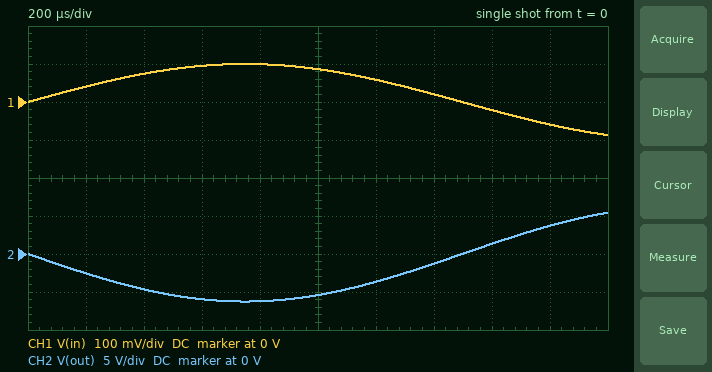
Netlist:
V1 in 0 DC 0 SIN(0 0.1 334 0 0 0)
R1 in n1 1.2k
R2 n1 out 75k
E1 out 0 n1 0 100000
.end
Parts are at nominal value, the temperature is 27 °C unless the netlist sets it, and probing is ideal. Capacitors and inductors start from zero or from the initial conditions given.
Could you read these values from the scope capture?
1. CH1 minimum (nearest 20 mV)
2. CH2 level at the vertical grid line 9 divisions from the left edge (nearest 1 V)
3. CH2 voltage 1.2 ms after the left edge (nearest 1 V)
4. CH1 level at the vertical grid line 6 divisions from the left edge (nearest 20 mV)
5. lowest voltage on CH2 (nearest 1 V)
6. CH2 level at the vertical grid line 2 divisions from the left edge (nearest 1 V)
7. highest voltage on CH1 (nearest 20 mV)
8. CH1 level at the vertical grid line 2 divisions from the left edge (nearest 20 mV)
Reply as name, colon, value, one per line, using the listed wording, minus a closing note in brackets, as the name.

CH1 minimum: -80 mV
CH2 level at the vertical grid line 9 divisions from the left edge: 4 V
CH2 voltage 1.2 ms after the left edge: -4 V
CH1 level at the vertical grid line 6 divisions from the left edge: 60 mV
lowest voltage on CH2: -6 V
CH2 level at the vertical grid line 2 divisions from the left edge: -5 V
highest voltage on CH1: 100 mV
CH1 level at the vertical grid line 2 divisions from the left edge: 80 mV
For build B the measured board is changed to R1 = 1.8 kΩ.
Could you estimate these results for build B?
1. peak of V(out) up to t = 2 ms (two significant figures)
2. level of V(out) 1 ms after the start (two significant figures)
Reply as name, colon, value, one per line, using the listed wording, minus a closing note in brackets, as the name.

peak of V(out) up to t = 2 ms: 3.6 V
level of V(out) 1 ms after the start: -3.6 V
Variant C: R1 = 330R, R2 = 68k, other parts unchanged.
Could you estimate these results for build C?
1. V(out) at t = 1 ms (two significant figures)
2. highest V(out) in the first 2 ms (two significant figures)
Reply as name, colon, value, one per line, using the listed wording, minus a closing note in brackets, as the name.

V(out) at t = 1 ms: -18 V
highest V(out) in the first 2 ms: 18 V
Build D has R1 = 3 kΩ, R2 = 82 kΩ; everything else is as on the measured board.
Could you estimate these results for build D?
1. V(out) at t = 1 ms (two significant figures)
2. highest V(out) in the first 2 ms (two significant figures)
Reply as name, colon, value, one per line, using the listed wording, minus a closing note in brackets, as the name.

V(out) at t = 1 ms: -2.4 V
highest V(out) in the first 2 ms: 2.4 V
